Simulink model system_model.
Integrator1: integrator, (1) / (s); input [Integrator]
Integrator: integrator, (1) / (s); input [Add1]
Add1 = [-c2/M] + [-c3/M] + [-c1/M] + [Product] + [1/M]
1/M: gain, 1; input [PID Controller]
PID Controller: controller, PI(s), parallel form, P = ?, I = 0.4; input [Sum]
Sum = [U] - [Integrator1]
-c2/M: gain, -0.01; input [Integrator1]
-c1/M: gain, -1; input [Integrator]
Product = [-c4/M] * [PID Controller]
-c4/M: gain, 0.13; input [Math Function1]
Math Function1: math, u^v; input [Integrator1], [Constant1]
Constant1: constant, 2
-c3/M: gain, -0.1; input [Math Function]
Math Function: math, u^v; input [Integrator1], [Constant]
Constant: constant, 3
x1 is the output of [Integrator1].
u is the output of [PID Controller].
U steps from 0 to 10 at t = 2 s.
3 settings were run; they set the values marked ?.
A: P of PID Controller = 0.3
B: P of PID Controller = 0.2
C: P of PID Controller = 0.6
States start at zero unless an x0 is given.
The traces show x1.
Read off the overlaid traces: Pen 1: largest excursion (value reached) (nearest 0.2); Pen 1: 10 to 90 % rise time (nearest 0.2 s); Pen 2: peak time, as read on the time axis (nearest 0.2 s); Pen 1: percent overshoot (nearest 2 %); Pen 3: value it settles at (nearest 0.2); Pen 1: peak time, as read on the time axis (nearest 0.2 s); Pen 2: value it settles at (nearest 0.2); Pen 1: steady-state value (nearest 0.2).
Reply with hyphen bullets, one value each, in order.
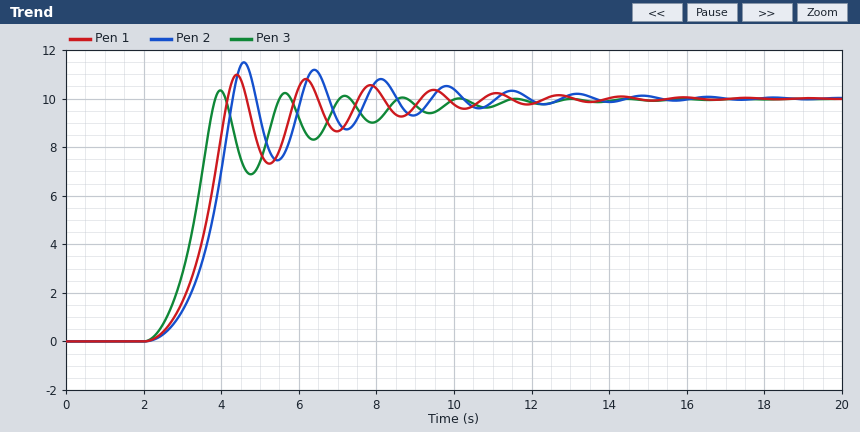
- 11.0
- 1.2 s
- 4.6 s
- 10 %
- 10.0
- 4.4 s
- 10.0
- 10.0
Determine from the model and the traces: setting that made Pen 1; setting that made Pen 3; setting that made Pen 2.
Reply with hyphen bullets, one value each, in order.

- A
- C
- B
